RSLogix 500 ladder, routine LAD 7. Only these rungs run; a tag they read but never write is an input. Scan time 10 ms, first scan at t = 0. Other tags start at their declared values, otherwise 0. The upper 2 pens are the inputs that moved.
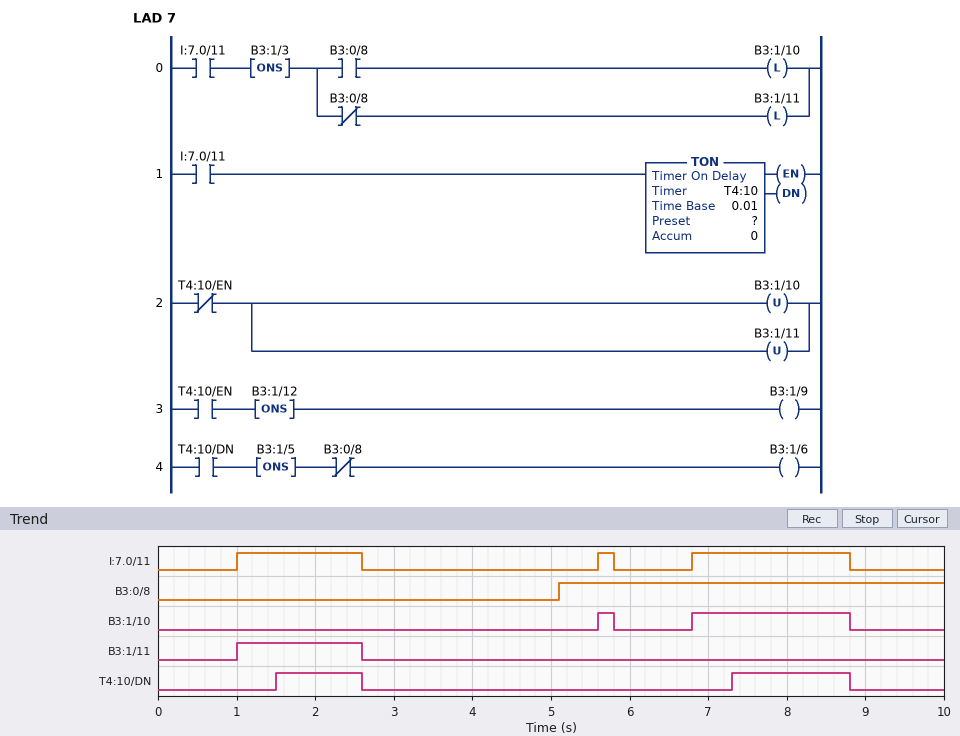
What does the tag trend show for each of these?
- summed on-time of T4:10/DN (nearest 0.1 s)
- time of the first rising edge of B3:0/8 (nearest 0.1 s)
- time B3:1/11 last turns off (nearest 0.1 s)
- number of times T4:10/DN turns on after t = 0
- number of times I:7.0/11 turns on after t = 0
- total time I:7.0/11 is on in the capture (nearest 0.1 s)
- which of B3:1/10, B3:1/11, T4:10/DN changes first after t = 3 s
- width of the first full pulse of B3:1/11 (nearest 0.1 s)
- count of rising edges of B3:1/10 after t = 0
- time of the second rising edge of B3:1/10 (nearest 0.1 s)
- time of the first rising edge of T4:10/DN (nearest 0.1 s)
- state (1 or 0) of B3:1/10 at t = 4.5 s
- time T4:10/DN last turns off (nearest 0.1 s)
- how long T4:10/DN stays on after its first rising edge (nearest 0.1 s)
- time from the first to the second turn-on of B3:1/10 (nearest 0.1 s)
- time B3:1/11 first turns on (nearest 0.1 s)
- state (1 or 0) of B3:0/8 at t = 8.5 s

2.6 s
5.1 s
2.6 s
2
3
3.8 s
B3:1/10
1.6 s
2
6.8 s
1.5 s
0
8.8 s
1.1 s
1.2 s
1.0 s
1
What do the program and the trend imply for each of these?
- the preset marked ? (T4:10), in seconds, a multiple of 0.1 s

0.5 s
